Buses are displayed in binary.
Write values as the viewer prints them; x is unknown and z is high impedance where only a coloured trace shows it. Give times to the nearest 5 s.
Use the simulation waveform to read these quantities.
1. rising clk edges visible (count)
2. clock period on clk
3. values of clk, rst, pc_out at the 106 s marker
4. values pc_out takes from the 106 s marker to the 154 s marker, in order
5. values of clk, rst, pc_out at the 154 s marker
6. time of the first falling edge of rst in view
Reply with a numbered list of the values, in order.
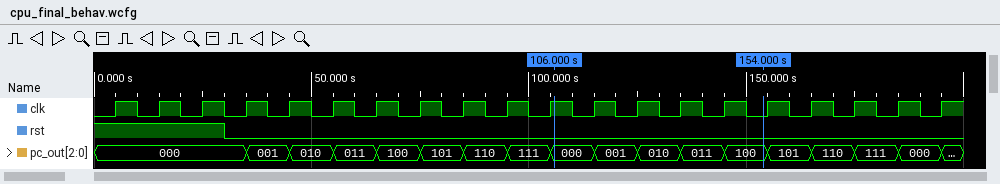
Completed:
1. 20
2. 10 s
3. clk=1, rst=0, pc_out=000
4. 000, 001, 010, 011, 100
5. clk=0, rst=0, pc_out=100
6. 30 s
